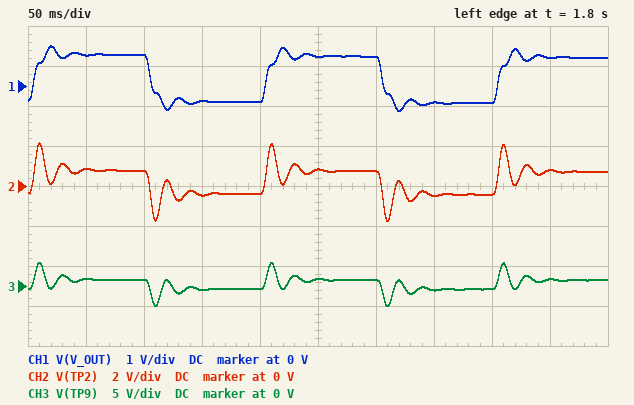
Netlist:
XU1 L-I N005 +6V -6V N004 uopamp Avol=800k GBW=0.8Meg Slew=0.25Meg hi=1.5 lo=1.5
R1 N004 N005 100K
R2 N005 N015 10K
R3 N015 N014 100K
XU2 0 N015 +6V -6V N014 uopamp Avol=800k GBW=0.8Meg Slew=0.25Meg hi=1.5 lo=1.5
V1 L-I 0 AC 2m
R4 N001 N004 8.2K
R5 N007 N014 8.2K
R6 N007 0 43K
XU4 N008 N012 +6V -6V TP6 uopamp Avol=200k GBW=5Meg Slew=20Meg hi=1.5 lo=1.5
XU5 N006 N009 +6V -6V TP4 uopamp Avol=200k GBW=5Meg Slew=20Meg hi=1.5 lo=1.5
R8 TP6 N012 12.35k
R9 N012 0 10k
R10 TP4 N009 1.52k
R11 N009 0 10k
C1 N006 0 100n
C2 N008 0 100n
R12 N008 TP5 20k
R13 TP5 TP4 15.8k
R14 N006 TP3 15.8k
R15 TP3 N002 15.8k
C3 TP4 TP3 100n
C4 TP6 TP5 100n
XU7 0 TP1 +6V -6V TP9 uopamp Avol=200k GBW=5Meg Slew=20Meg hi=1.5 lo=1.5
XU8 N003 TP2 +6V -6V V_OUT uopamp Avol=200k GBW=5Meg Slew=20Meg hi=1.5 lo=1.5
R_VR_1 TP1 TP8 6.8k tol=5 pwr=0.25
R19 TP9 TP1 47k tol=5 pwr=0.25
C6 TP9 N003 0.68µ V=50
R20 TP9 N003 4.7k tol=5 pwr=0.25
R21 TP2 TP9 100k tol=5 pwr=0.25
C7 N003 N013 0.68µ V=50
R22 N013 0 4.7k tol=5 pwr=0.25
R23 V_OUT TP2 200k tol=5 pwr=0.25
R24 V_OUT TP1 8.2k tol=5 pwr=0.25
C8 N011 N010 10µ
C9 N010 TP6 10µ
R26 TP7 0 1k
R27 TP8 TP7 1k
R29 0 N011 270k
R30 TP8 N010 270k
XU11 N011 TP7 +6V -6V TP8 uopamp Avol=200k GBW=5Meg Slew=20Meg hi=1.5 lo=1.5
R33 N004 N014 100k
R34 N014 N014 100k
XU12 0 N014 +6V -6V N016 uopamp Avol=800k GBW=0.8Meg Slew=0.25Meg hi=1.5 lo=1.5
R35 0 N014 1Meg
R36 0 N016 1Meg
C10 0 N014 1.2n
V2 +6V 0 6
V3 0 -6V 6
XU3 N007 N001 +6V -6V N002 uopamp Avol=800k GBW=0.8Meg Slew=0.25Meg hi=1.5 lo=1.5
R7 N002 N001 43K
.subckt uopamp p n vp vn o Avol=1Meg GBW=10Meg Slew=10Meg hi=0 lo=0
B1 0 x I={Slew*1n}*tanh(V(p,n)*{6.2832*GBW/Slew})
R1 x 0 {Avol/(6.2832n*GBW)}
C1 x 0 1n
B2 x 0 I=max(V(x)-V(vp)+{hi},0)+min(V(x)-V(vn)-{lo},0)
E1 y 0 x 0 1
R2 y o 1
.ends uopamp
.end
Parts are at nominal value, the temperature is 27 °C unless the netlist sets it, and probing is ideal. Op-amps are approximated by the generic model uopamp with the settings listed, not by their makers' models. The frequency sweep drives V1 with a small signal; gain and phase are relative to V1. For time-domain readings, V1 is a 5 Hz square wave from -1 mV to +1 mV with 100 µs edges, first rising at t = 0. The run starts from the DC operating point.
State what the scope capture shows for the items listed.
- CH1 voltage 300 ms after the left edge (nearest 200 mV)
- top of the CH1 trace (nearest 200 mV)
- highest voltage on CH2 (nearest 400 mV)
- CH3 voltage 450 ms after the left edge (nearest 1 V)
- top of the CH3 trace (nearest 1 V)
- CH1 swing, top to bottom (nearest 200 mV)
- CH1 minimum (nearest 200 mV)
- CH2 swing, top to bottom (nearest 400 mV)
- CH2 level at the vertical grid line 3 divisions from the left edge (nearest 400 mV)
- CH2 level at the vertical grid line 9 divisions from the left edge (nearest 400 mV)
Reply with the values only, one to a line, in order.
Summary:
800 mV
1.0 V
2.0 V
1 V
3 V
1.6 V
-600 mV
4.0 V
-400 mV
800 mV
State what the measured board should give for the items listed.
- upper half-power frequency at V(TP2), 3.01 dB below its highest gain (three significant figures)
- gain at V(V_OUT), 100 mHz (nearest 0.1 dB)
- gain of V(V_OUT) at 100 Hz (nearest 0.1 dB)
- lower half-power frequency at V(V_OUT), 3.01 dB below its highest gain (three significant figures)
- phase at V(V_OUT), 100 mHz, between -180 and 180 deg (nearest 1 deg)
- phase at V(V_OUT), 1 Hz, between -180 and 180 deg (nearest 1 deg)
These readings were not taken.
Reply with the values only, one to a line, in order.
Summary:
61.6 Hz
56.4 dB
49.2 dB
50.4 mHz
42 deg
1 deg
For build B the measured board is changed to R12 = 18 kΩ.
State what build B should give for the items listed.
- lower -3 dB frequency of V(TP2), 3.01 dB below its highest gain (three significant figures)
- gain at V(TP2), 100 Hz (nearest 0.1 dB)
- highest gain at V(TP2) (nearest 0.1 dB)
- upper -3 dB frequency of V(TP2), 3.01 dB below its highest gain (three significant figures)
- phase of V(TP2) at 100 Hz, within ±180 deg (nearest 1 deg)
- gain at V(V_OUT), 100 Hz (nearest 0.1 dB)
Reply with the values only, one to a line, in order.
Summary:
39.3 Hz
54.9 dB
68.3 dB
62.1 Hz
136 deg
50.5 dB
